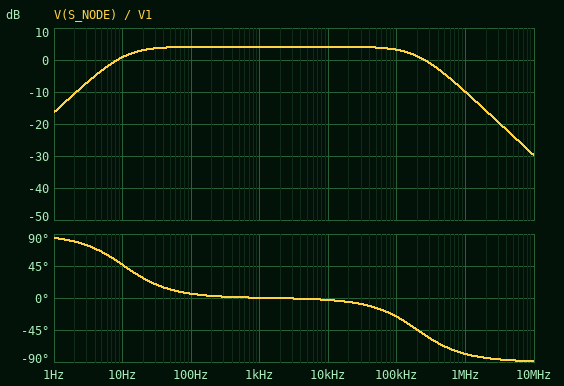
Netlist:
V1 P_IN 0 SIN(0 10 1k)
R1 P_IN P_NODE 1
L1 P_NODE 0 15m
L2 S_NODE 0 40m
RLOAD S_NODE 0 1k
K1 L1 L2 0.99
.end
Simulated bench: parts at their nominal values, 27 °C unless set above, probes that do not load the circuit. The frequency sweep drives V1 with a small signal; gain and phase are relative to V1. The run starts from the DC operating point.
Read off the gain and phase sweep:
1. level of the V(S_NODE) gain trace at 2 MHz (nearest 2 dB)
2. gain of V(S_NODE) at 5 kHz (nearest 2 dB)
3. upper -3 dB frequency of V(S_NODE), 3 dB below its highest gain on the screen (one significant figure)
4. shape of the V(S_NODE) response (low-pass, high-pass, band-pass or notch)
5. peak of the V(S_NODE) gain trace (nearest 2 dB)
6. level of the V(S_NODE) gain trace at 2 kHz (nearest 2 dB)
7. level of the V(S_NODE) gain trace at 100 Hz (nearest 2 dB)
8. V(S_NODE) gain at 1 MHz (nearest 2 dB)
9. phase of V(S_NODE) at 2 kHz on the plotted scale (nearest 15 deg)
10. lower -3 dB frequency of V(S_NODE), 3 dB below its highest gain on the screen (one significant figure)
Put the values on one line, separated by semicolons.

-16 dB; 4 dB; 200 kHz; band-pass; 4 dB; 4 dB; 4 dB; -10 dB; 0 deg; 10 Hz
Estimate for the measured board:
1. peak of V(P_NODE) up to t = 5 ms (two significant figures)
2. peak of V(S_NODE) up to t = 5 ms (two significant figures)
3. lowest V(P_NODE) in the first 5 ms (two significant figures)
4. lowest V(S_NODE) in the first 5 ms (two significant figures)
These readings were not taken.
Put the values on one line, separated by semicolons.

9.9 V; 16 V; -10 V; -16 V
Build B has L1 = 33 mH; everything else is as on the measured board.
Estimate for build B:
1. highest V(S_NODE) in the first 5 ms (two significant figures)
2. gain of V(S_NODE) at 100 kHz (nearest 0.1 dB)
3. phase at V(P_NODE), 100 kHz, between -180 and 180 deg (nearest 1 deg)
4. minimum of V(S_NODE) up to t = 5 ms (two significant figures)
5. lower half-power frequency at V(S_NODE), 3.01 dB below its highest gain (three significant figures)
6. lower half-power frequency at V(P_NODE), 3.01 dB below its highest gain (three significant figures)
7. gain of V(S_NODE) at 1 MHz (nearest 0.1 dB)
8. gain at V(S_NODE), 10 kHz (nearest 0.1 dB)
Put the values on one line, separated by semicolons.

11 V; -0.2 dB; 0 deg; -11 V; 4.82 Hz; 4.83 Hz; -13.4 dB; 0.7 dB
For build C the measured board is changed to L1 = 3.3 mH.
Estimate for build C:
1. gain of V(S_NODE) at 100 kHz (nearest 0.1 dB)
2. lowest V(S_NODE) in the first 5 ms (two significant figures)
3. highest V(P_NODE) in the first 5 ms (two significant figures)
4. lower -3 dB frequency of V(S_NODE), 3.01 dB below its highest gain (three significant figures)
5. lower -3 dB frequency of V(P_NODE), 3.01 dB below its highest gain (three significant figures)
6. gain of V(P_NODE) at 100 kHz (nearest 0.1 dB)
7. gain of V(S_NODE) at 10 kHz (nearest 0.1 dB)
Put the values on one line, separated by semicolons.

9.7 dB; -35 V; 9.7 V; 47.6 Hz; 48.8 Hz; -0.1 dB; 10.6 dB
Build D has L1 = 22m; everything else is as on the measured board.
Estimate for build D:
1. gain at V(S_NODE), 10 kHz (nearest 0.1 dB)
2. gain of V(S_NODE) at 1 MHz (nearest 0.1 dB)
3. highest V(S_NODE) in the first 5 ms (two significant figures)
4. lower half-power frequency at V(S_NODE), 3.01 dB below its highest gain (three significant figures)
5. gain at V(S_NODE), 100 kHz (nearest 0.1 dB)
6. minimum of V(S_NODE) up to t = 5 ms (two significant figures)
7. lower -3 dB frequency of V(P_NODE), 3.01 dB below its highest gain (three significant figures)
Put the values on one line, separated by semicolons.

2.5 dB; -11.6 dB; 13 V; 7.22 Hz; 1.5 dB; -13 V; 7.25 Hz
